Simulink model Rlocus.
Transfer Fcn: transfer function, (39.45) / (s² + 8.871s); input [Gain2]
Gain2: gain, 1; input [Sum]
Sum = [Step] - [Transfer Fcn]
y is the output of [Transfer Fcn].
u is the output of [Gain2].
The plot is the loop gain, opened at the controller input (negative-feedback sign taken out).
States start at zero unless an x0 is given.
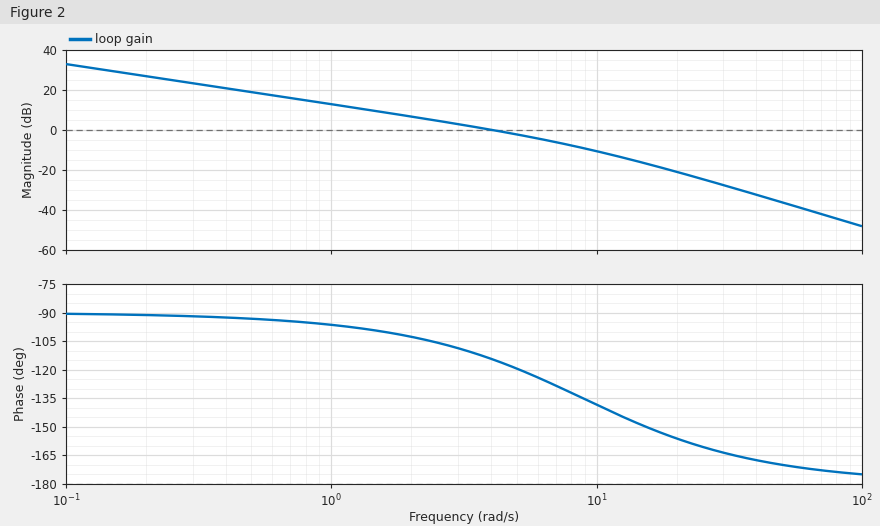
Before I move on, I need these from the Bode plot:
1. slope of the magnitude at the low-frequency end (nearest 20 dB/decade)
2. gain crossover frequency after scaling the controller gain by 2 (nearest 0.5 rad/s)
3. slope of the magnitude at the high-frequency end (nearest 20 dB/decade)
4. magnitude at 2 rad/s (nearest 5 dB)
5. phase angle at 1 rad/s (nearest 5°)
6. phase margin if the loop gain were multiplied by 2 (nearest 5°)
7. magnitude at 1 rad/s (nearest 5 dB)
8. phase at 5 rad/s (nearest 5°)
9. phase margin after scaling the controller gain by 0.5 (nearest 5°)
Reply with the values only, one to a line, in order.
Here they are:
-20 dB/decade
7.0 rad/s
-40 dB/decade
5 dB
-95°
50°
15 dB
-120°
75°
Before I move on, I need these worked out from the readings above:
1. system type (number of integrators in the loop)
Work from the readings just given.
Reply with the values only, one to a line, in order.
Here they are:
1
